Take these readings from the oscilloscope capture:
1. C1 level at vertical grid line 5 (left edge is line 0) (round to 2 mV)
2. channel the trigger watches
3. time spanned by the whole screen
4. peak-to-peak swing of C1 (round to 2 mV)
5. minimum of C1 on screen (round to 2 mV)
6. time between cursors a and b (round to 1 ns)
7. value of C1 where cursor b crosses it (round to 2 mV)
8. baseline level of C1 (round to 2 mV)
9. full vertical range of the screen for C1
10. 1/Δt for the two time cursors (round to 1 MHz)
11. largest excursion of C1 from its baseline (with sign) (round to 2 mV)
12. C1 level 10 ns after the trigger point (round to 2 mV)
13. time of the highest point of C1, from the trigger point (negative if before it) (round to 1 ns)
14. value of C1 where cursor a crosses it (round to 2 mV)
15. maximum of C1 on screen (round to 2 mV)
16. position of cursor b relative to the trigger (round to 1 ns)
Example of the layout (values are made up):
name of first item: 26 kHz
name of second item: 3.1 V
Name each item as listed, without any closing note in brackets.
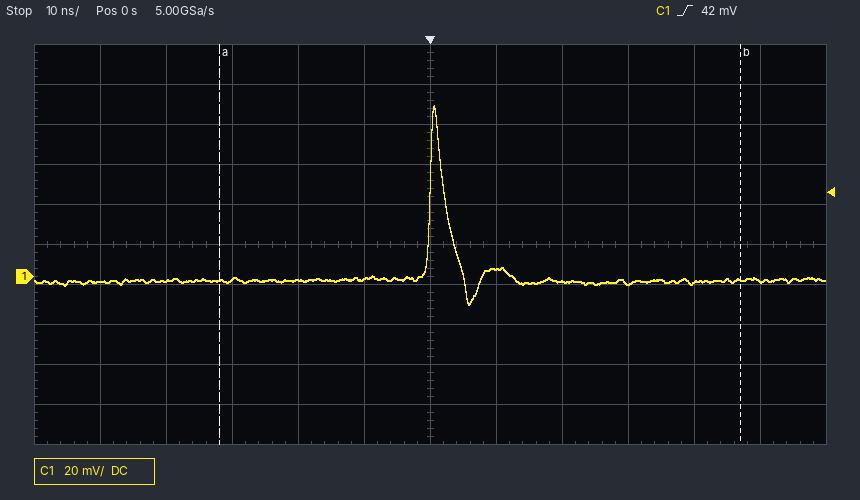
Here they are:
C1 level at vertical grid line 5 (left edge is line 0): -2 mV
channel the trigger watches: C1
time spanned by the whole screen: 120 ns
peak-to-peak swing of C1: 100 mV
minimum of C1 on screen: -14 mV
time between cursors a and b: 79 ns
value of C1 where cursor b crosses it: -2 mV
baseline level of C1: -2 mV
full vertical range of the screen for C1: 200 mV
1/Δt for the two time cursors: 13 MHz
largest excursion of C1 from its baseline (with sign): +88 mV
C1 level 10 ns after the trigger point: 4 mV
time of the highest point of C1, from the trigger point (negative if before it): +1 ns
value of C1 where cursor a crosses it: -2 mV
maximum of C1 on screen: 86 mV
position of cursor b relative to the trigger: +47 ns
